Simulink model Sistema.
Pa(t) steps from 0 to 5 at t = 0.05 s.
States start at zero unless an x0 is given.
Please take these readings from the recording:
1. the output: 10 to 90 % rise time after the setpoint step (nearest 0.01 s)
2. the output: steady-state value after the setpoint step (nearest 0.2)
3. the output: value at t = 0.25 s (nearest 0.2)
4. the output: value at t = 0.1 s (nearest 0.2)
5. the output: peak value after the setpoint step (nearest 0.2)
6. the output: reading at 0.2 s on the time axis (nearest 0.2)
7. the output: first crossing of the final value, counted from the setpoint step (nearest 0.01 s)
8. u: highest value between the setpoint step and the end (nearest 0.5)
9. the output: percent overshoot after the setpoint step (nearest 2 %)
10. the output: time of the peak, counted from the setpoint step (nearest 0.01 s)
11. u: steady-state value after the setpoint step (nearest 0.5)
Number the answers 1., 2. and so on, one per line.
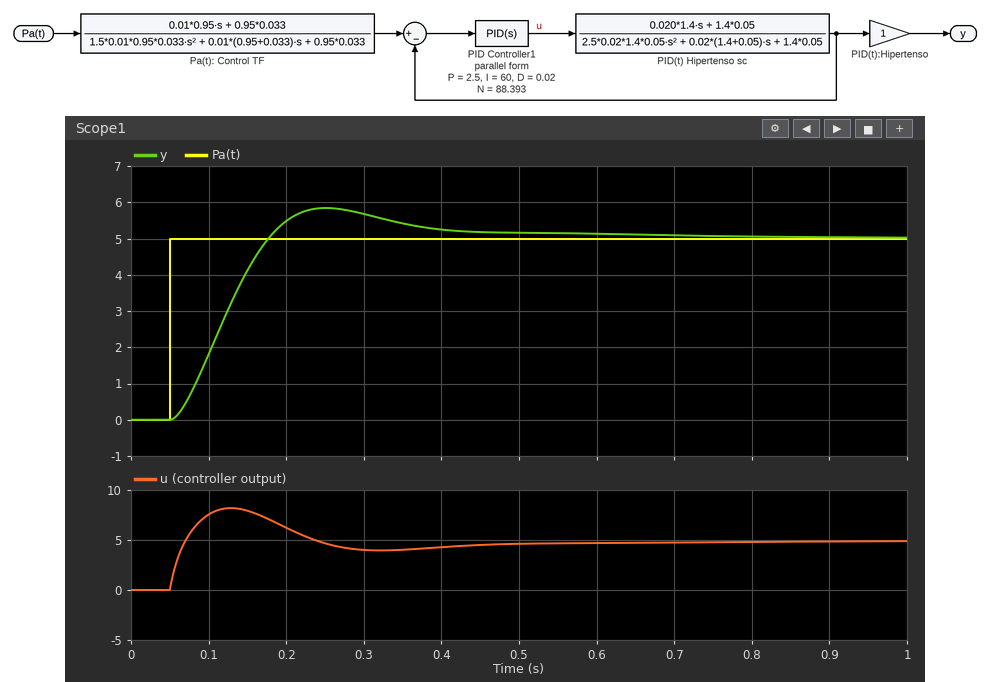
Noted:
1. 0.09 s
2. 5.0
3. 5.8
4. 1.8
5. 5.8
6. 5.4
7. 0.13 s
8. 8.0
9. 16 %
10. 0.20 s
11. 5.0
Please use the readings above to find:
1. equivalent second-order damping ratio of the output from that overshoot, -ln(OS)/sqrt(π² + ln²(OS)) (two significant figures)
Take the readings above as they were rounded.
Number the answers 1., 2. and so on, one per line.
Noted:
1. 0.50
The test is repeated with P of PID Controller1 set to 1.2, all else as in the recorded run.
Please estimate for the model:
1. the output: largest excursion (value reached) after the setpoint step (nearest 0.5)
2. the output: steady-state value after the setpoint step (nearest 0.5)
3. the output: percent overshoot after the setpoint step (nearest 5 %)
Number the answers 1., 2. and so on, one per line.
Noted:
1. 6.5
2. 5.0
3. 25 %
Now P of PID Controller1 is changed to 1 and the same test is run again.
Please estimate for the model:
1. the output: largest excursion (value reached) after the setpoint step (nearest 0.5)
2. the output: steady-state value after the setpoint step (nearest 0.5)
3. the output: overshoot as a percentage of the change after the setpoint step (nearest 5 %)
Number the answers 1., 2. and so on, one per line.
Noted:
1. 6.5
2. 5.0
3. 30 %
